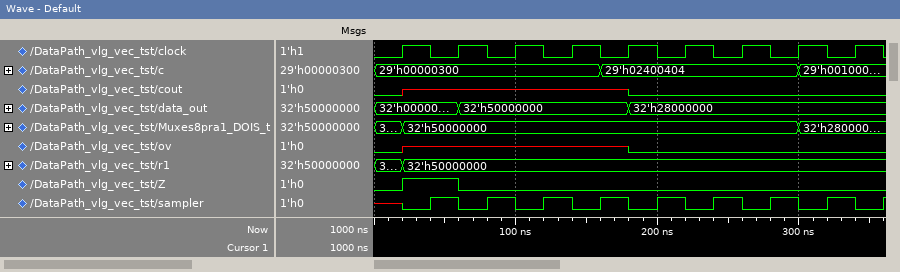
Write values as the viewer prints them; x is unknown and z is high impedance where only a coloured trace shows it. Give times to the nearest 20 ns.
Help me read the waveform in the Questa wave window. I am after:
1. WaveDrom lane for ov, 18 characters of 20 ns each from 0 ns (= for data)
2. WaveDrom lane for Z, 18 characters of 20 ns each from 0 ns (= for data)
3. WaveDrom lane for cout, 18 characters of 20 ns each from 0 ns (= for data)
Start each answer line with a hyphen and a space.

- {name: 'ov', wave: '0x.......0........'}
- {name: 'Z', wave: '01.0..............'}
- {name: 'cout', wave: '0x.......0........'}
